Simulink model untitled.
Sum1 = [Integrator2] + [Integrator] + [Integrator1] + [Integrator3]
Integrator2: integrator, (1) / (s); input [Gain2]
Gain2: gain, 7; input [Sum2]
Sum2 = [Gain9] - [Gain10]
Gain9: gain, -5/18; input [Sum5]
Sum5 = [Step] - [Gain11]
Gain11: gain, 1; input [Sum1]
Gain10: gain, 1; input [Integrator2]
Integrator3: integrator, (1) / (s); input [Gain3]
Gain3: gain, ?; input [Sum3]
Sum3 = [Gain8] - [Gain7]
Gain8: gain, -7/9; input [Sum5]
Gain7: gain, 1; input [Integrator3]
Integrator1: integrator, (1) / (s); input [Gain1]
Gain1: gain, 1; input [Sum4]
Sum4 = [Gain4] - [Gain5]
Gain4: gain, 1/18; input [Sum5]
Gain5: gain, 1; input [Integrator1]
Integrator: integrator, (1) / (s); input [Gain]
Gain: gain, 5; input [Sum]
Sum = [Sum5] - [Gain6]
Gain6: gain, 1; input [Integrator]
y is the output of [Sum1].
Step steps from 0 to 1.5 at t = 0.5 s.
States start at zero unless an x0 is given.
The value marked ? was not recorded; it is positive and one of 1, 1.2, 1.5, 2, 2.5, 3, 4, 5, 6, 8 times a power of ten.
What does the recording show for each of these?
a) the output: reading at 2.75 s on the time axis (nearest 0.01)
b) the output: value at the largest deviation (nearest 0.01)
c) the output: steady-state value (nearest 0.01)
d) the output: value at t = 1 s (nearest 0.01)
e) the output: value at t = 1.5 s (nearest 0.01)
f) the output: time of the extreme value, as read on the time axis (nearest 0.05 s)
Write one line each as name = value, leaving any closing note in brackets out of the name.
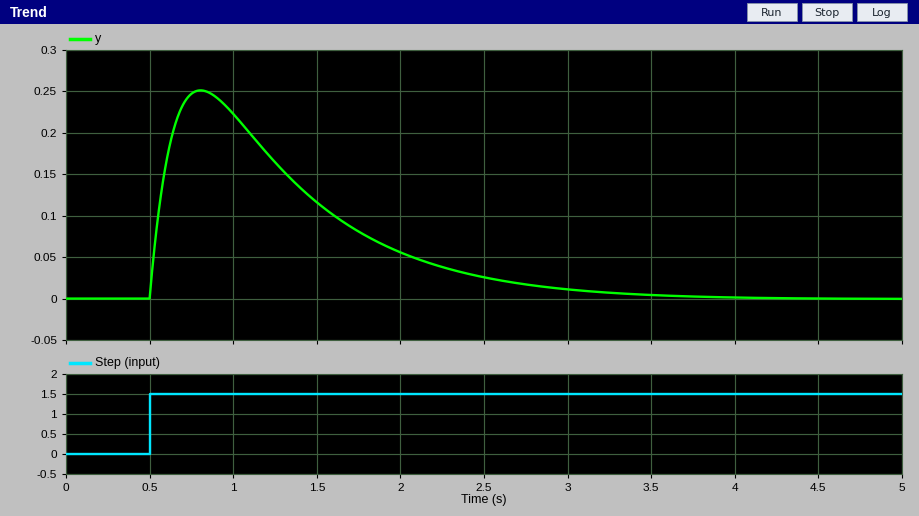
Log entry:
the output: reading at 2.75 s on the time axis = 0.02
the output: value at the largest deviation = 0.25
the output: steady-state value = 0.00
the output: value at t = 1 s = 0.22
the output: value at t = 1.5 s = 0.12
the output: time of the extreme value, as read on the time axis = 0.80 s
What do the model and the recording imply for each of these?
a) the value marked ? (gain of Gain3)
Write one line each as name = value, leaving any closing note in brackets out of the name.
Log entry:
the value marked ? = 2
